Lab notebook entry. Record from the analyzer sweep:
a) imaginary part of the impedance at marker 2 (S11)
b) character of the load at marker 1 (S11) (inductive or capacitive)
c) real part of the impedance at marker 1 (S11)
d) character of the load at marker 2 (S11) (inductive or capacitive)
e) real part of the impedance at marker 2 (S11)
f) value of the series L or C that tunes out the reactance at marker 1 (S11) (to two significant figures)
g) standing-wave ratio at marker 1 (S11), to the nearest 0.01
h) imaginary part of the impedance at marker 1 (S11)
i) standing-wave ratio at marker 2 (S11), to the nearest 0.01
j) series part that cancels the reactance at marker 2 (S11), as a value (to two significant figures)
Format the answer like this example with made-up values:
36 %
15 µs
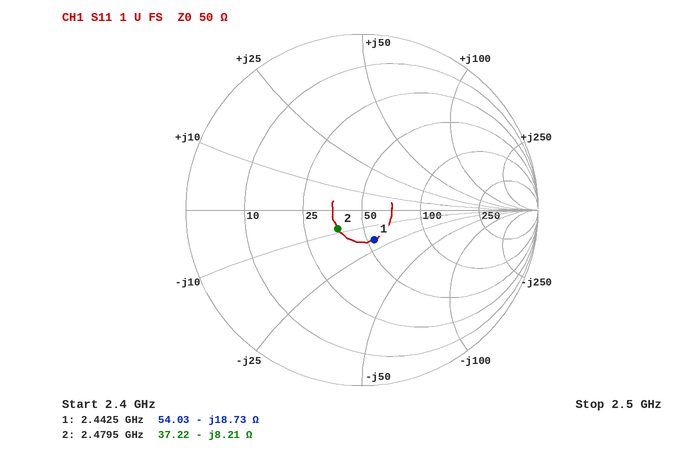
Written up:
-8.21 Ω
capacitive
54.03 Ω
capacitive
37.22 Ω
1.2 nH
1.44
-18.73 Ω
1.42
530 pH
